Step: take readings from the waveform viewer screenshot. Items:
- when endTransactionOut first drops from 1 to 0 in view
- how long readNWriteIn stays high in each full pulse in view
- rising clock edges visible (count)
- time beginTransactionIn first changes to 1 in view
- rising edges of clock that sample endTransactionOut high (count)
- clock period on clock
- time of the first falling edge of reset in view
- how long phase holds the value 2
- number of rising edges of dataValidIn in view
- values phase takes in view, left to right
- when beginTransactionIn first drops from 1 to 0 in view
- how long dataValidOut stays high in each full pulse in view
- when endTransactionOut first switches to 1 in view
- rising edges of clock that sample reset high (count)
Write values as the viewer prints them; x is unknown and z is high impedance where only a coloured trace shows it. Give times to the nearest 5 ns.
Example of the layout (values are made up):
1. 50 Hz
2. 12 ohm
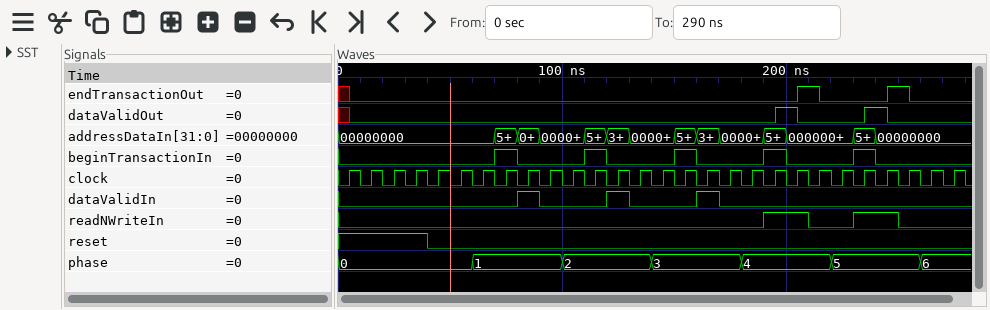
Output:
1. 215 ns
2. 20 ns, 20 ns
3. 28
4. 70 ns
5. 2
6. 10 ns
7. 40 ns
8. 40 ns
9. 3
10. 0, 1, 2, 3, 4, 5, 6
11. 80 ns
12. 10 ns, 10 ns
13. 205 ns
14. 4
